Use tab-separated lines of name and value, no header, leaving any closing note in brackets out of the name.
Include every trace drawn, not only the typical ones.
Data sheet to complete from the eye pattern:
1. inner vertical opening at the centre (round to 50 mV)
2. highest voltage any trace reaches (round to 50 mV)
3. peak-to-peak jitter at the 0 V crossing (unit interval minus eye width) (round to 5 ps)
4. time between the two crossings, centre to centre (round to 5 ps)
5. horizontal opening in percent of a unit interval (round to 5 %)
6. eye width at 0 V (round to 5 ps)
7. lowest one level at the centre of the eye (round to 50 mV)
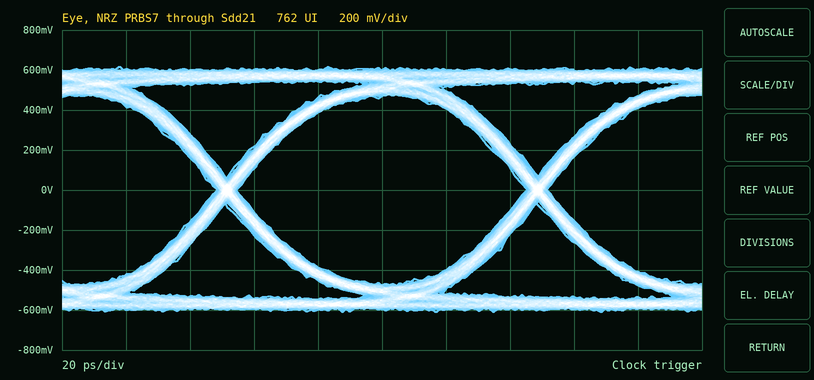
inner vertical opening at the centre	950 mV
highest voltage any trace reaches	600 mV
peak-to-peak jitter at the 0 V crossing (unit interval minus eye width)	5 ps
time between the two crossings, centre to centre	95 ps
horizontal opening in percent of a unit interval	95 %
eye width at 0 V	90 ps
lowest one level at the centre of the eye	450 mV
